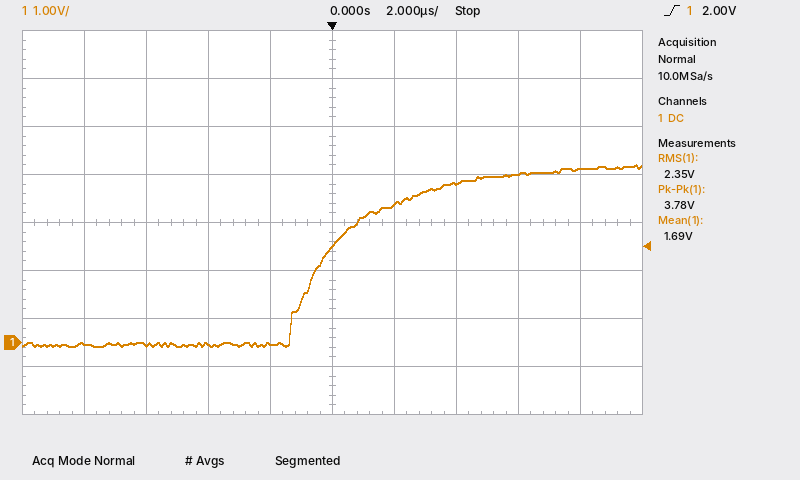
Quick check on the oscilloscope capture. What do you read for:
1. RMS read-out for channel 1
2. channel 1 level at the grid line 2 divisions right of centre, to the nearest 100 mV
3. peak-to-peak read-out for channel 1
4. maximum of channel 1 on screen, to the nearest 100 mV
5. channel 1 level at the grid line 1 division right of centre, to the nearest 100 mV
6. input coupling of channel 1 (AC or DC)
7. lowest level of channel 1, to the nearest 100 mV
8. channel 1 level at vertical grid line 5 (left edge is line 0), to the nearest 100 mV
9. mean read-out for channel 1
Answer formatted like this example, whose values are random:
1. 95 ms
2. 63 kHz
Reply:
1. 2.35 V
2. 3.3 V
3. 3.78 V
4. 3.7 V
5. 2.9 V
6. DC
7. -100 mV
8. 2.0 V
9. 1.69 V
